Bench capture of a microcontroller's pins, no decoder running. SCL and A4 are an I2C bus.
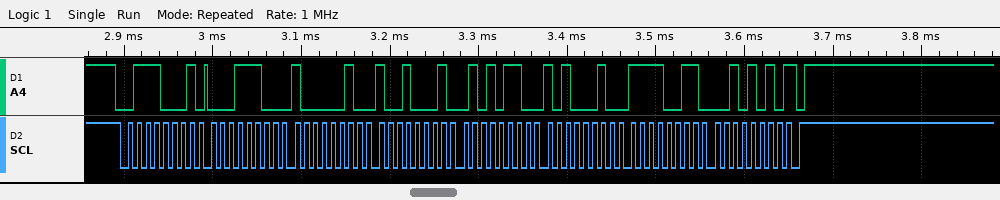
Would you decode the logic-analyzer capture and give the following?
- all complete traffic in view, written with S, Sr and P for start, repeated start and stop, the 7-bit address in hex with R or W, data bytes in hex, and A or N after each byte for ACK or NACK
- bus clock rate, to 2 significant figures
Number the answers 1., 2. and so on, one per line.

1. S 38R A 1C A 82 A 91 A 56 A A2 A F3 A 2A N P
2. 100 kHz
